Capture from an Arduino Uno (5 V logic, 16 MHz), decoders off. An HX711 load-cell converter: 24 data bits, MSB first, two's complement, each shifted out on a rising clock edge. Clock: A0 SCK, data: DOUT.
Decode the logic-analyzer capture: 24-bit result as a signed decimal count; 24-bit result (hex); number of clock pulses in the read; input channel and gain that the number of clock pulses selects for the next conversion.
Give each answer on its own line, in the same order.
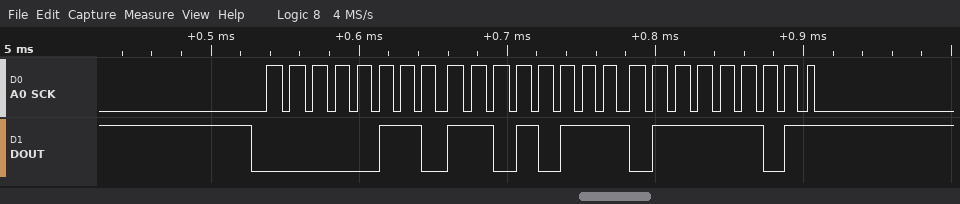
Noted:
448381
0x06D77D
25
channel A, gain 128
